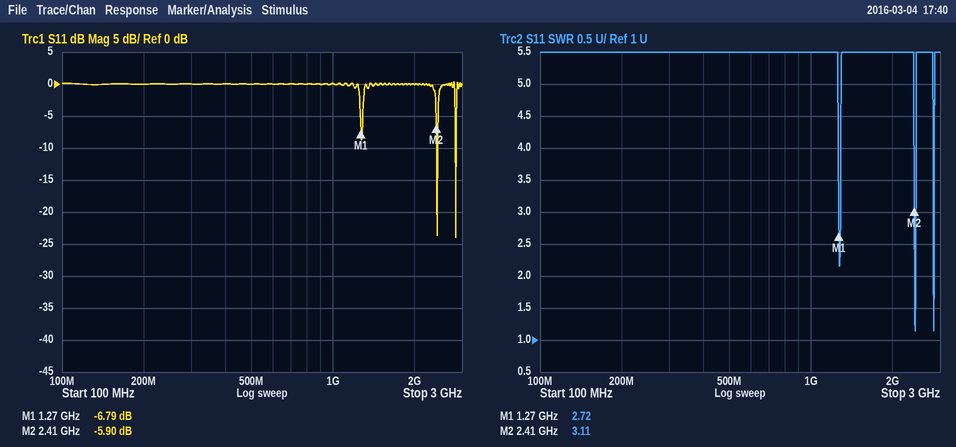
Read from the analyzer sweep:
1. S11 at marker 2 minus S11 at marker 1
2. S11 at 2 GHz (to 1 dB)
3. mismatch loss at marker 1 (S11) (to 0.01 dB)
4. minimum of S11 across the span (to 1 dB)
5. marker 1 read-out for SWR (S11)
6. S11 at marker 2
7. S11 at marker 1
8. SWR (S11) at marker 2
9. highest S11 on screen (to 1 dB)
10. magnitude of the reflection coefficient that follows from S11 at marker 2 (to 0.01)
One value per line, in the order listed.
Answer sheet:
0.89 dB
0 dB
1.02 dB
-24 dB
2.72
-5.90 dB
-6.79 dB
3.11
0 dB
0.51
